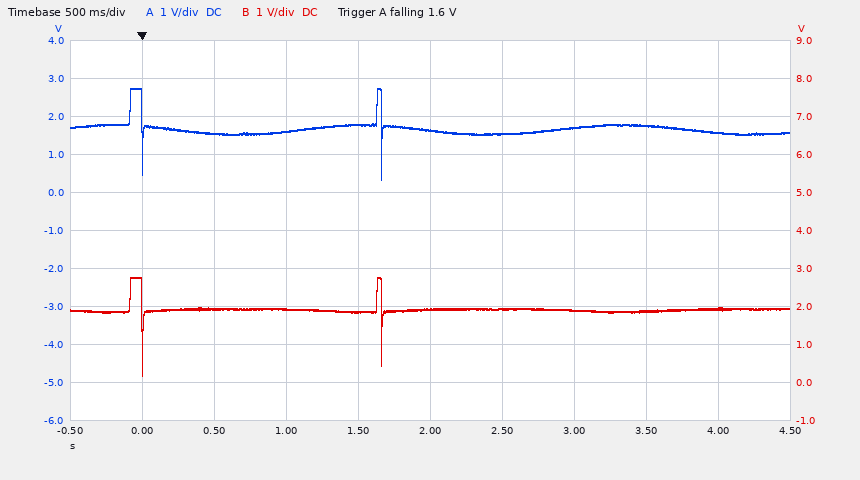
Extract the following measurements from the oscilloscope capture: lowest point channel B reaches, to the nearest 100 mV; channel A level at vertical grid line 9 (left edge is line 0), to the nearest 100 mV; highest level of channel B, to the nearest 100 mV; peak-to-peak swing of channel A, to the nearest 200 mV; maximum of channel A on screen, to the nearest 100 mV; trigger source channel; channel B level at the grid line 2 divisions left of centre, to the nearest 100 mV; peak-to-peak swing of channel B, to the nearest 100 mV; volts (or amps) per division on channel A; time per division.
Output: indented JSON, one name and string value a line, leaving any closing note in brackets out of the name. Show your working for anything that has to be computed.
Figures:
{
  "lowest point channel B reaches, to the nearest 100 mV": "200 mV",
  "channel A level at vertical grid line 9 (left edge is line 0), to the nearest 100 mV": "1.6 V",
  "highest level of channel B, to the nearest 100 mV": "2.8 V",
  "peak-to-peak swing of channel A, to the nearest 200 mV": "2.4 V",
  "maximum of channel A on screen, to the nearest 100 mV": "2.7 V",
  "trigger source channel": "channel A",
  "channel B level at the grid line 2 divisions left of centre, to the nearest 100 mV": "1.9 V",
  "peak-to-peak swing of channel B, to the nearest 100 mV": "2.8 V − (200 mV) = 2.6 V",
  "volts (or amps) per division on channel A": "1 V",
  "time per division": "500 ms"
}
